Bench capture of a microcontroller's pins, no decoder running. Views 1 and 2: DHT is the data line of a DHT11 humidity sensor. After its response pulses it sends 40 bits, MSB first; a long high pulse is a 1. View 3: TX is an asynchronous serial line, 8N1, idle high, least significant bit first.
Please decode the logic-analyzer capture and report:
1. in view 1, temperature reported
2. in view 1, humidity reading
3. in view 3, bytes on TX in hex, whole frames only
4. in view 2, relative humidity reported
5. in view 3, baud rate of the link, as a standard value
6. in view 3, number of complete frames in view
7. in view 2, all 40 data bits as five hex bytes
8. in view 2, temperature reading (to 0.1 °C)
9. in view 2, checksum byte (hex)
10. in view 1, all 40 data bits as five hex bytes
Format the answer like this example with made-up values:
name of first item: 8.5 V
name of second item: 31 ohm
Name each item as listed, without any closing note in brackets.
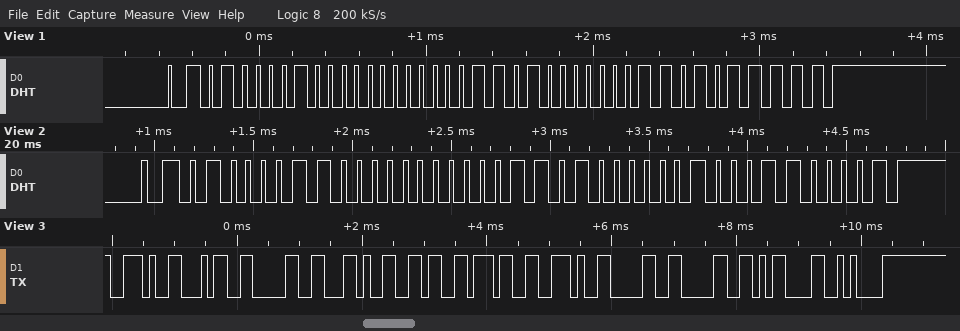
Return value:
in view 1, temperature reported: 26.3 °C
in view 1, humidity reading: 66 %
in view 3, bytes on TX in hex, whole frames only: 2E 34 30 2C 36 37 2E 30 30 0D 0A
in view 2, relative humidity reported: 67 %
in view 3, baud rate of the link, as a standard value: 9600 baud
in view 3, number of complete frames in view: 11
in view 2, all 40 data bits as five hex bytes: 43 00 1A 04 61
in view 2, temperature reading: 26.4 °C
in view 2, checksum byte: 0x61
in view 1, all 40 data bits as five hex bytes: 42 00 1A 03 5F
